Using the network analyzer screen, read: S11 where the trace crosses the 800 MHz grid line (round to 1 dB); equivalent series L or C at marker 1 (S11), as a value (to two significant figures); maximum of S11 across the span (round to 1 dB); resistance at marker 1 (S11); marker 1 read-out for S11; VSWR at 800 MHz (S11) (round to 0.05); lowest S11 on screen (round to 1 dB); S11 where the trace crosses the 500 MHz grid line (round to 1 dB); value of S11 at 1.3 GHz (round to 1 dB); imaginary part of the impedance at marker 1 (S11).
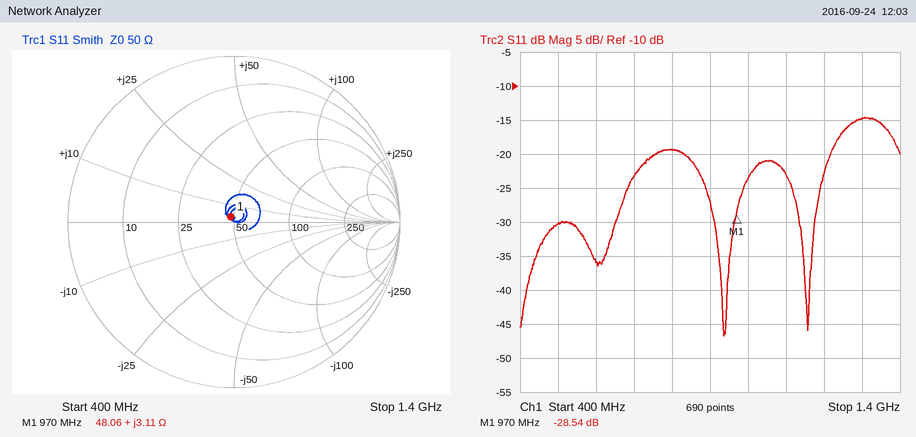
-19 dB
510 pH
-15 dB
48.06 Ω
-28.54 dB
1.25
-47 dB
-30 dB
-15 dB
+3.11 Ω
